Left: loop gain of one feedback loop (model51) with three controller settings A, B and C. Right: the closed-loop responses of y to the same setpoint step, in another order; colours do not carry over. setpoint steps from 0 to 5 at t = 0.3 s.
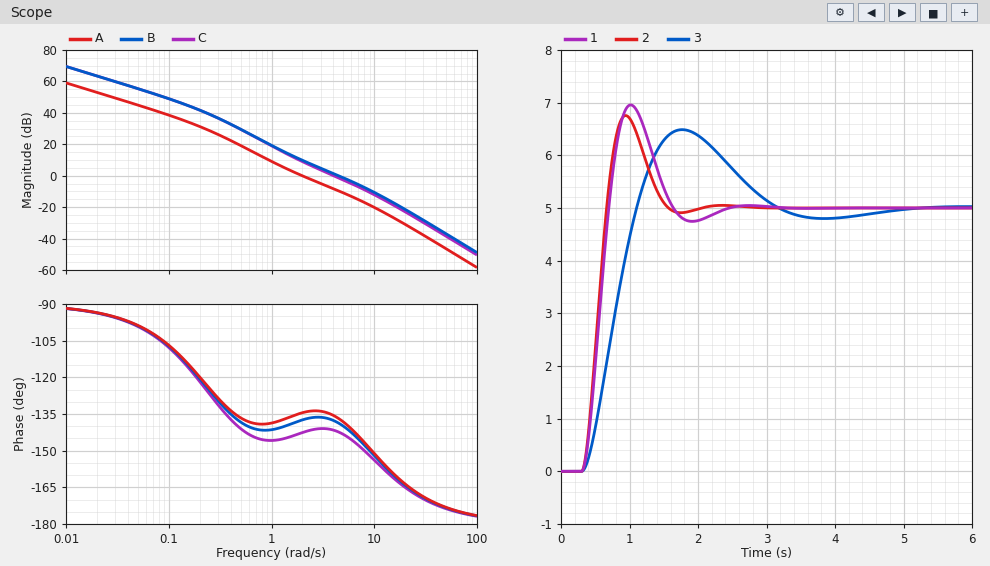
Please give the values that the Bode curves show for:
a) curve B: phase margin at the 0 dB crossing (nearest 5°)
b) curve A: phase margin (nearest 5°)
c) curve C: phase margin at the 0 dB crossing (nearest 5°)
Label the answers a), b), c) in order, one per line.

a) 40°
b) 45°
c) 40°
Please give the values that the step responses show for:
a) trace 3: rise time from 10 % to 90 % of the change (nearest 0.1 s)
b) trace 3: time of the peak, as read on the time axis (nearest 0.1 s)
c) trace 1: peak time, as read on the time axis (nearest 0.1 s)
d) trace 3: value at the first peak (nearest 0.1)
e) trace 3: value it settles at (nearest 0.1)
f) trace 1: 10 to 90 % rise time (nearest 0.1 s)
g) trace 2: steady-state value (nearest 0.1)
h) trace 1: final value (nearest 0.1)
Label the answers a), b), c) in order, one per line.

a) 0.6 s
b) 1.8 s
c) 1.0 s
d) 6.5
e) 5.0
f) 0.3 s
g) 5.0
h) 5.0
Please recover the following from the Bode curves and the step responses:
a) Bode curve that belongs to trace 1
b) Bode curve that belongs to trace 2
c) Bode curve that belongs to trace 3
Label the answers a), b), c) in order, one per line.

a) C
b) B
c) A
